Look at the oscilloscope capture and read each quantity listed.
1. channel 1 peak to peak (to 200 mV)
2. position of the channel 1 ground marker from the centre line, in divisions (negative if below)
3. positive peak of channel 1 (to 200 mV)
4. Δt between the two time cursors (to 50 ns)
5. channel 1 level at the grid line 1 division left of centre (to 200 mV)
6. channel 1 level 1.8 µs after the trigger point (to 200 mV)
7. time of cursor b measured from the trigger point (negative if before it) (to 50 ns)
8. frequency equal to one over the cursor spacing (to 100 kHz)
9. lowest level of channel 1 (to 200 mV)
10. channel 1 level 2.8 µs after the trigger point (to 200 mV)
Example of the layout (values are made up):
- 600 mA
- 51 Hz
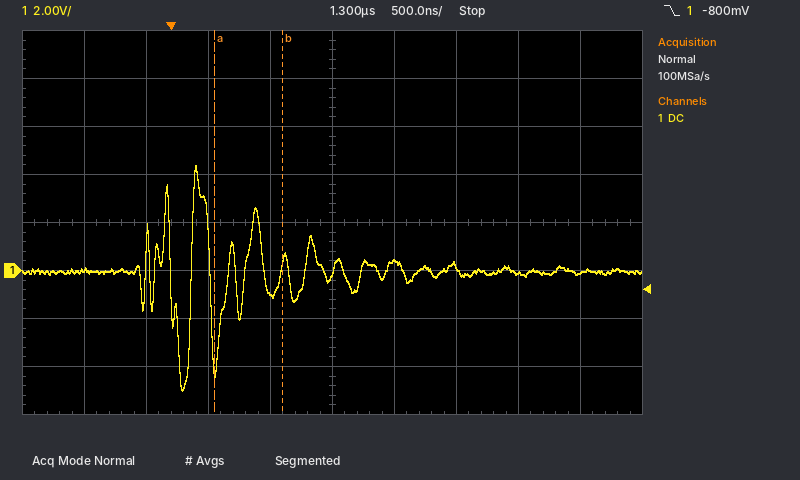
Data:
- 9.4 V
- -1.0 div
- 4.4 V
- 550 ns
- -1.0 V
- 400 mV
- +900 ns
- 1.8 MHz
- -5.0 V
- -200 mV
